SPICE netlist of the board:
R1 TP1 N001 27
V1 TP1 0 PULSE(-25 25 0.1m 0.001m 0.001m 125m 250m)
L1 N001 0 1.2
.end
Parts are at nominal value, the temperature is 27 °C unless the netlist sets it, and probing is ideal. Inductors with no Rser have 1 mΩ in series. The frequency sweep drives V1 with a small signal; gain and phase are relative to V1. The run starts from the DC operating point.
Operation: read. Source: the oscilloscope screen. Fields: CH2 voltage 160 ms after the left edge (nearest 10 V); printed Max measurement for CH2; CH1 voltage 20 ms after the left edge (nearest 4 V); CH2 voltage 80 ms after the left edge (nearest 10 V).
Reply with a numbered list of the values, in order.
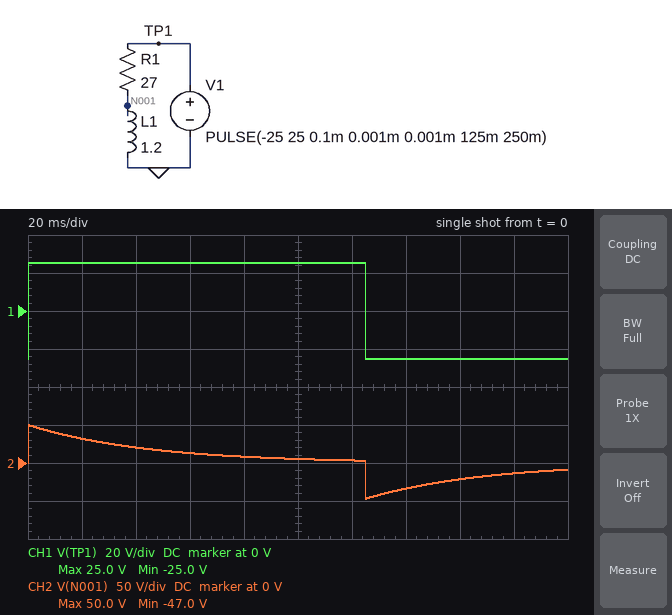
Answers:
1. -20 V
2. 50.0 V
3. 24 V
4. 10 V
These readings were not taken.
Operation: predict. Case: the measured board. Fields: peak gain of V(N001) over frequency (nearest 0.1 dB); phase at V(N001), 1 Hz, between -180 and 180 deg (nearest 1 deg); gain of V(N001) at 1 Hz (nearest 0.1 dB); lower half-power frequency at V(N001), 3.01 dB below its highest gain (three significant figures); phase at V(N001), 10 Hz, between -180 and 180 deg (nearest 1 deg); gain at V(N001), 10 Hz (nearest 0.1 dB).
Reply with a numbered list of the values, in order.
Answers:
1. 0 dB
2. 74 deg
3. -11.4 dB
4. 3.58 Hz
5. 20 deg
6. -0.5 dB
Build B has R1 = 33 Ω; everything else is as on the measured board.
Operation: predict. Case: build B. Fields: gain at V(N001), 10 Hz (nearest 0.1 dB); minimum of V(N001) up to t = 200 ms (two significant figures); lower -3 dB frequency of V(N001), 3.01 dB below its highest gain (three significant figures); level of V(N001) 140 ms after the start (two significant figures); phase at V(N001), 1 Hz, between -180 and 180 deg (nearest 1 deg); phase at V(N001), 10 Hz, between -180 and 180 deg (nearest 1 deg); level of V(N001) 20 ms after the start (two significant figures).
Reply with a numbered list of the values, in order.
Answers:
1. -0.8 dB
2. -48 V
3. 4.38 Hz
4. -32 V
5. 77 deg
6. 24 deg
7. 29 V
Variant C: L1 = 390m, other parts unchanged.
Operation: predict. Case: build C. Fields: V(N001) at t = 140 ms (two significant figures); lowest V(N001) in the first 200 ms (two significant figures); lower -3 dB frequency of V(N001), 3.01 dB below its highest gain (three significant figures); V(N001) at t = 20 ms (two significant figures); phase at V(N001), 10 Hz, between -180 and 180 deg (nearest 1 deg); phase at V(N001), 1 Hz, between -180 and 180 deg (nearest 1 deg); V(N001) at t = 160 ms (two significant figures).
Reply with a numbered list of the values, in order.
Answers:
1. -18 V
2. -50 V
3. 11.0 Hz
4. 13 V
5. 48 deg
6. 85 deg
7. -4.5 V
